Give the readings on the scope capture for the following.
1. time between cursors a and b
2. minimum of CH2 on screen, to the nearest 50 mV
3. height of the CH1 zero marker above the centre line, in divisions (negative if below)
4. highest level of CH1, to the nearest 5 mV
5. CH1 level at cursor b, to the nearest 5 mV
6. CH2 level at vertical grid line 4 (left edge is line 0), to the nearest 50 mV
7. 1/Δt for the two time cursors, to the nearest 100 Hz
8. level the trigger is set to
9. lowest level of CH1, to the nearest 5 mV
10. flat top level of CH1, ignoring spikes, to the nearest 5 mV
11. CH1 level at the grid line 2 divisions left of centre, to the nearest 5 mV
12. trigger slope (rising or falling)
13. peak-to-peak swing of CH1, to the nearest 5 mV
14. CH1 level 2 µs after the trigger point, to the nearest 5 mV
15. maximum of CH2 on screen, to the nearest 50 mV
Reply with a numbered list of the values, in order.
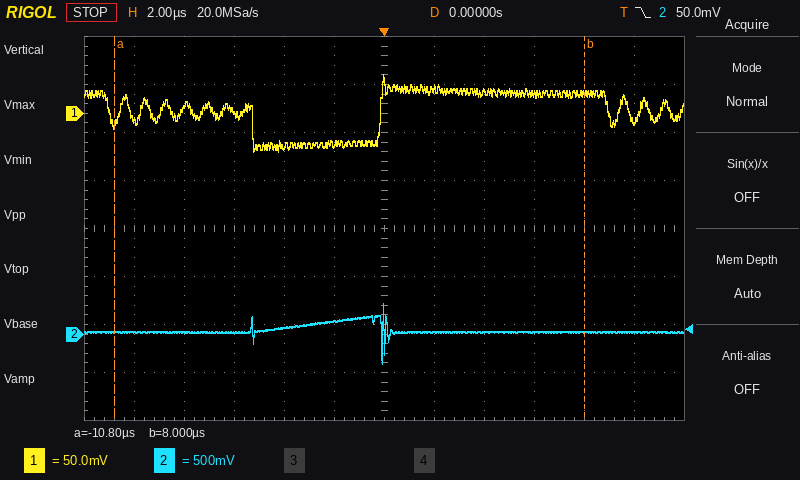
1. 18.8 µs
2. -300 mV
3. +2.4 div
4. 40 mV
5. 20 mV
6. 50 mV
7. 53.2 kHz
8. 50.0 mV
9. -40 mV
10. 20 mV
11. -35 mV
12. falling
13. 80 mV
14. 25 mV
15. 300 mV
